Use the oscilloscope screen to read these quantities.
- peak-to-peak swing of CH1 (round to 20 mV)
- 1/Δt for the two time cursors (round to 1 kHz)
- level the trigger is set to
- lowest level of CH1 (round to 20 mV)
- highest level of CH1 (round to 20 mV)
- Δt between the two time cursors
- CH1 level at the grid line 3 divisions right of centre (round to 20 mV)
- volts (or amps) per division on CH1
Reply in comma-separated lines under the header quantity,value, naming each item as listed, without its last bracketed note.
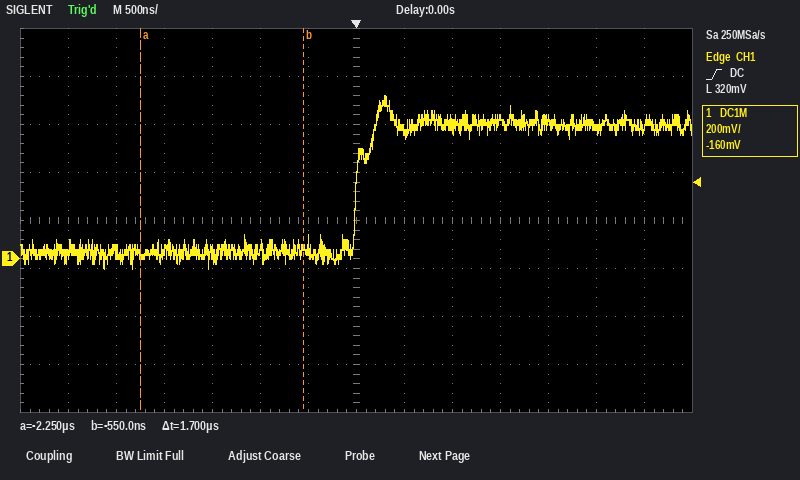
quantity,value
peak-to-peak swing of CH1,720 mV
1/Δt for the two time cursors,588 kHz
level the trigger is set to,320 mV
lowest level of CH1,-40 mV
highest level of CH1,680 mV
Δt between the two time cursors,1.7 µs
CH1 level at the grid line 3 divisions right of centre,580 mV
volts (or amps) per division on CH1,200 mV
